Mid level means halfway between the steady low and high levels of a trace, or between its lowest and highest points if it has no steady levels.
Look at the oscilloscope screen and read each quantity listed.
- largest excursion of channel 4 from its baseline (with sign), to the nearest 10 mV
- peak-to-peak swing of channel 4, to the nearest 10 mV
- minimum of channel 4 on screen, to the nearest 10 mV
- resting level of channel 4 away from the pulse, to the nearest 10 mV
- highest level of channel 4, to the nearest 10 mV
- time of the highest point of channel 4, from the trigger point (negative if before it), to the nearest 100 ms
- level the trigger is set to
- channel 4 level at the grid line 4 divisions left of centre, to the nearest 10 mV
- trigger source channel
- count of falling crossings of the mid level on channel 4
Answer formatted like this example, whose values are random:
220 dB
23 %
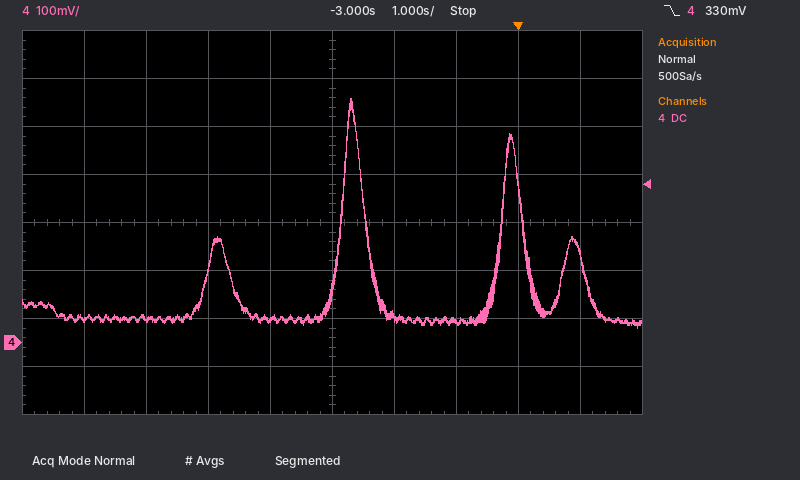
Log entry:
+460 mV
480 mV
30 mV
50 mV
510 mV
-2.7 s
330 mV
50 mV
channel 4
2
